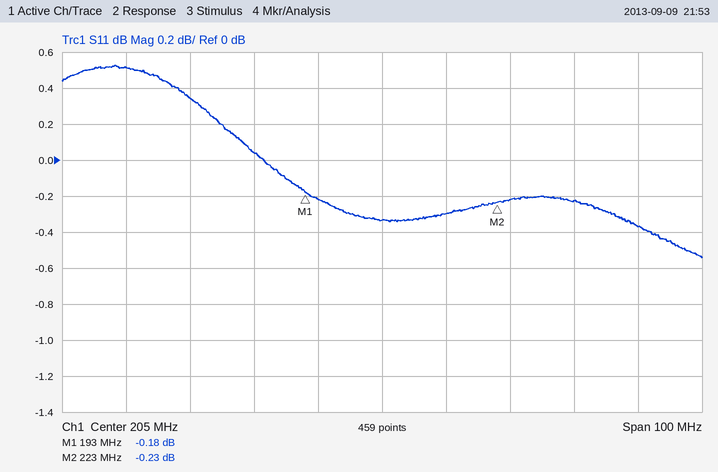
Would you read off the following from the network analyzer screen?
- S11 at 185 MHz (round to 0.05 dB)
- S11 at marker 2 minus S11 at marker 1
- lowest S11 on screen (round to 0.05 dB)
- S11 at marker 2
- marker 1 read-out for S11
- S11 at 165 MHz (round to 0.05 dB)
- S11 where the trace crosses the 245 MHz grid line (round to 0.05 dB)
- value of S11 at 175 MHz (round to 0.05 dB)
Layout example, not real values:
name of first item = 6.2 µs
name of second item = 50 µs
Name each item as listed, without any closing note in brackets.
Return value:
S11 at 185 MHz = 0.05 dB
S11 at marker 2 minus S11 at marker 1 = -0.05 dB
lowest S11 on screen = -0.55 dB
S11 at marker 2 = -0.23 dB
marker 1 read-out for S11 = -0.18 dB
S11 at 165 MHz = 0.50 dB
S11 where the trace crosses the 245 MHz grid line = -0.35 dB
value of S11 at 175 MHz = 0.35 dB
